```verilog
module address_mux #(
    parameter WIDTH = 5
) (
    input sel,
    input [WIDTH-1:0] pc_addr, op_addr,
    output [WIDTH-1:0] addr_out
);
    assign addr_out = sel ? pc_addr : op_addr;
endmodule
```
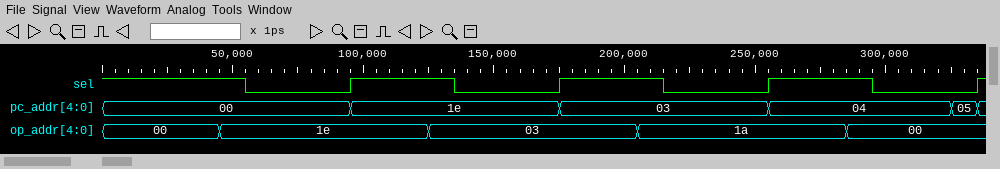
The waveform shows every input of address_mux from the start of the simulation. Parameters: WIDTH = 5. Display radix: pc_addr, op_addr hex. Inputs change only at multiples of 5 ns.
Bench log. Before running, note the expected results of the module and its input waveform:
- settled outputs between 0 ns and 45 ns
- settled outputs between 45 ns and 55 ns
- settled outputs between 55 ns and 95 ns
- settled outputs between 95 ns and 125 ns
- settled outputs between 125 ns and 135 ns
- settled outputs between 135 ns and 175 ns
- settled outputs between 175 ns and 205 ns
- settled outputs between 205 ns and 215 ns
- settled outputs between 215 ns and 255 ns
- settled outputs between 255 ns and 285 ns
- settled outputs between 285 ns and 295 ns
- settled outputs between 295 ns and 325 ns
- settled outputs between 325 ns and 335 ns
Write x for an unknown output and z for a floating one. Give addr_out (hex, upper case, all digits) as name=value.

addr_out=00
addr_out=00
addr_out=1E
addr_out=1E
addr_out=1E
addr_out=03
addr_out=03
addr_out=03
addr_out=1A
addr_out=04
addr_out=04
addr_out=00
addr_out=00
